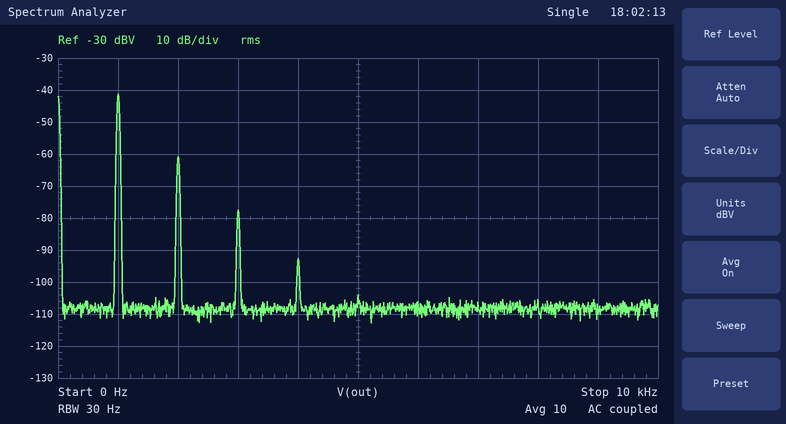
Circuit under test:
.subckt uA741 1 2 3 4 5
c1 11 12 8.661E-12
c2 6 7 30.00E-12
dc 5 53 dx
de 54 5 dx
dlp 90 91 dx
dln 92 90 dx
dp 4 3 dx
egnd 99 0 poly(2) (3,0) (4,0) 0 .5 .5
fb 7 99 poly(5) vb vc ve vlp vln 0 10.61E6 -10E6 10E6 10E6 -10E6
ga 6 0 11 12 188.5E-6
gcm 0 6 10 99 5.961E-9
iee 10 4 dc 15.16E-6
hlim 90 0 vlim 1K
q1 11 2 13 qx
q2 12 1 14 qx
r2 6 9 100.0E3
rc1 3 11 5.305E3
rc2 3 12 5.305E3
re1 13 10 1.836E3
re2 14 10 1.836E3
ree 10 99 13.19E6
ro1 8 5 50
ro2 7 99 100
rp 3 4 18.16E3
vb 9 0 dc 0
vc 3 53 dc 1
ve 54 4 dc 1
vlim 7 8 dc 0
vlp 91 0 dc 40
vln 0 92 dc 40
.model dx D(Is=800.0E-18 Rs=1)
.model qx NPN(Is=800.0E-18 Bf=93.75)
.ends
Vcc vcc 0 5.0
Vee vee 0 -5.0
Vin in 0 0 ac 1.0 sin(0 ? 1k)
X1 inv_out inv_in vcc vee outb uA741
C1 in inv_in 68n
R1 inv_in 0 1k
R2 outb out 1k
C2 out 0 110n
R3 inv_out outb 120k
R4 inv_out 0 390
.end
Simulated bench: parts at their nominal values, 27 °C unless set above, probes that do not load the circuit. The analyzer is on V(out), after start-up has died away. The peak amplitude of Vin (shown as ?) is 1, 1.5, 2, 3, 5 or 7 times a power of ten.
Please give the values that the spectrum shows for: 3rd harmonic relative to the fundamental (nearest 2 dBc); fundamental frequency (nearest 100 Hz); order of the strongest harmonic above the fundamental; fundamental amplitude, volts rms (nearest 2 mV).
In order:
-36 dBc
1.0 kHz
2
8 mV
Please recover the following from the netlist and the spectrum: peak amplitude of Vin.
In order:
20 mV
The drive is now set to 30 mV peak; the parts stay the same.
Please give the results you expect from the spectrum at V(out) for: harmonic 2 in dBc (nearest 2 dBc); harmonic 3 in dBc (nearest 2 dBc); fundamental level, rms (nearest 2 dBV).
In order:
-14 dBc
-26 dBc
-36 dBV
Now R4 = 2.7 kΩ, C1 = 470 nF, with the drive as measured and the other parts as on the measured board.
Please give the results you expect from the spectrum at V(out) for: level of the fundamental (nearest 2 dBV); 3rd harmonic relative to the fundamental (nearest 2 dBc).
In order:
-60 dBV
-44 dBc
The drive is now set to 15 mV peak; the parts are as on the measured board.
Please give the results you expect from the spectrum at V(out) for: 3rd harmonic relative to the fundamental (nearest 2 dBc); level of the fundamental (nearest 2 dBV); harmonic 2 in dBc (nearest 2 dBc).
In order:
-42 dBc
-44 dBV
-22 dBc
